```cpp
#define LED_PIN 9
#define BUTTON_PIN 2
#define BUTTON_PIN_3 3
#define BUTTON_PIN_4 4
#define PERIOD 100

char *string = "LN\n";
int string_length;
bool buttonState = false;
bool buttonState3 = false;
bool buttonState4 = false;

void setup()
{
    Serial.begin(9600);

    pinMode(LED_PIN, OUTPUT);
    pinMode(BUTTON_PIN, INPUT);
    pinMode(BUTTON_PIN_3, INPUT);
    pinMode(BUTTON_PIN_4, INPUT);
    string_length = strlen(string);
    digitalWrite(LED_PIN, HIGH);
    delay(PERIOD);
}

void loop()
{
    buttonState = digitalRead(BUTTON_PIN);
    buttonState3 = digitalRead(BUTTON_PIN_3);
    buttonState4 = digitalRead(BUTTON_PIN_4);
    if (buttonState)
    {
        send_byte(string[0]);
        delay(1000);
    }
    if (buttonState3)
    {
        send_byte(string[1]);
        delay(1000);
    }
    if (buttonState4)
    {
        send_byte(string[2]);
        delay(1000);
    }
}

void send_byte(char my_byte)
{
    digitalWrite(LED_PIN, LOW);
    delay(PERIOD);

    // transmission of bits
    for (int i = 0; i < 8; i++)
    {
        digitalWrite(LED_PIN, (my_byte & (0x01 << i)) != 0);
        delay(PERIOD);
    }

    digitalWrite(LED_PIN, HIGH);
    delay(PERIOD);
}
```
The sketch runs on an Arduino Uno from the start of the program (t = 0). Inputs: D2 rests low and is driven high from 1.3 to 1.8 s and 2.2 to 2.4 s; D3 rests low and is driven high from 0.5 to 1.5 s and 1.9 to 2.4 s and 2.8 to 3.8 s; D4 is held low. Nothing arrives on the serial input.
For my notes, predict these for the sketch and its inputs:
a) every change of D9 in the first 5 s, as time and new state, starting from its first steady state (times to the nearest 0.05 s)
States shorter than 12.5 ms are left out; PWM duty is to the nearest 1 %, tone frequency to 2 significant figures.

0 s high; 0.5 s low; 0.7 s high; 1 s low; 1.2 s high; 1.3 s low; 1.4 s high; 2.8 s low; 3 s high; 3.3 s low; 3.5 s high; 3.6 s low; 3.7 s high
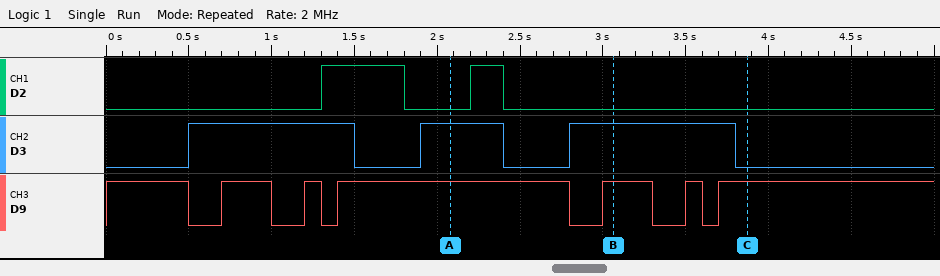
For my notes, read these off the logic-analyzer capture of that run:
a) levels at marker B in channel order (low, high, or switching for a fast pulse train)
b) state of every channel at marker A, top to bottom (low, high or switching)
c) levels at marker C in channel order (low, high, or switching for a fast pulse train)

D2 low, D3 high, D9 high
D2 low, D3 high, D9 high
D2 low, D3 low, D9 high
